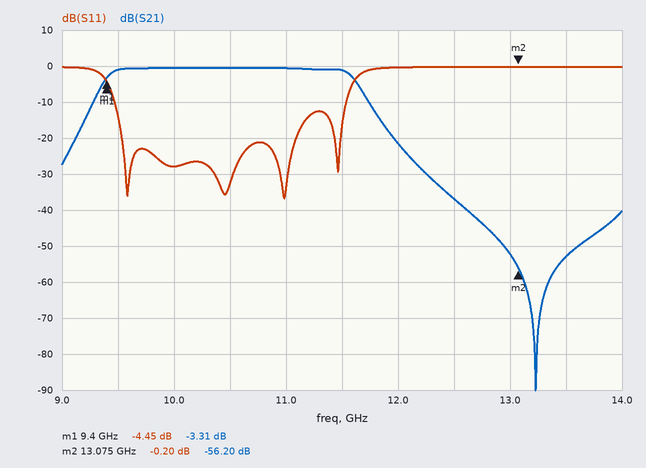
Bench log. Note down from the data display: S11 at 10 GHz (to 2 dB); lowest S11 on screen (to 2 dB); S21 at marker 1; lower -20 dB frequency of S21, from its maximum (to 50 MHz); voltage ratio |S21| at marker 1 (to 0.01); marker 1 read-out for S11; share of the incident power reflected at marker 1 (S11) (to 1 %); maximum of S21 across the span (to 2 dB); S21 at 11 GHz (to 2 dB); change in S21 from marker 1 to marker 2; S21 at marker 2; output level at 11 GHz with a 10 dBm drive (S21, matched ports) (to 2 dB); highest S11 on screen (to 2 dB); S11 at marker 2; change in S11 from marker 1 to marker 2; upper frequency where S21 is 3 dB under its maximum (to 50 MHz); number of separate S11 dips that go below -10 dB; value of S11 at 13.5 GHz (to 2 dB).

-28 dB
-36 dB
-3.31 dB
9.10 GHz
0.68
-4.45 dB
36 %
0 dB
0 dB
-52.89 dB
-56.20 dB
10 dBm
0 dB
-0.20 dB
4.25 dB
11.60 GHz
4
0 dB
